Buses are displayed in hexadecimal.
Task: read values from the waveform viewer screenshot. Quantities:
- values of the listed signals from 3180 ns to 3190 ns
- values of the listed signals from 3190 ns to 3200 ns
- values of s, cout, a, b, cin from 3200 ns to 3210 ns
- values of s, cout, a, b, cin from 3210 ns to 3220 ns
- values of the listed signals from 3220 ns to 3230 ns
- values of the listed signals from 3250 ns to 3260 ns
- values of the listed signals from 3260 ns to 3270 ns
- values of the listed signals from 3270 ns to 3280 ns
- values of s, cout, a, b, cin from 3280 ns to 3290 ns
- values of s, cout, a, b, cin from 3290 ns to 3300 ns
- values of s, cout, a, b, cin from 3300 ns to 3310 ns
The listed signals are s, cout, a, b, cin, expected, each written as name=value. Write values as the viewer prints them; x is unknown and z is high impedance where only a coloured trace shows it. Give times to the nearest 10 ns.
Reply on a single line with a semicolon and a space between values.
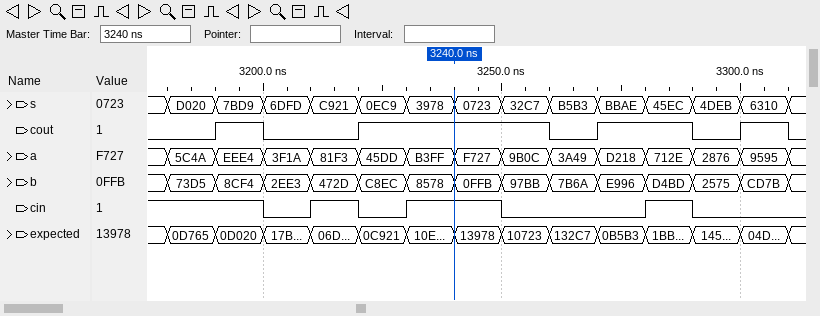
s=D020, cout=0, a=5C4A, b=73D5, cin=1, expected=0D765; s=7BD9, cout=1, a=EEE4, b=8CF4, cin=1, expected=0D020; s=6DFD, cout=0, a=3F1A, b=2EE3, cin=0; s=C921, cout=0, a=81F3, b=472D, cin=1; s=0EC9, cout=1, a=45DD, b=C8EC, cin=0, expected=0C921; s=32C7, cout=1, a=9B0C, b=97BB, cin=0, expected=10723; s=B5B3, cout=0, a=3A49, b=7B6A, cin=0, expected=132C7; s=BBAE, cout=1, a=D218, b=E996, cin=0, expected=0B5B3; s=45EC, cout=1, a=712E, b=D4BD, cin=1; s=4DEB, cout=0, a=2876, b=2575, cin=0; s=6310, cout=1, a=9595, b=CD7B, cin=0
